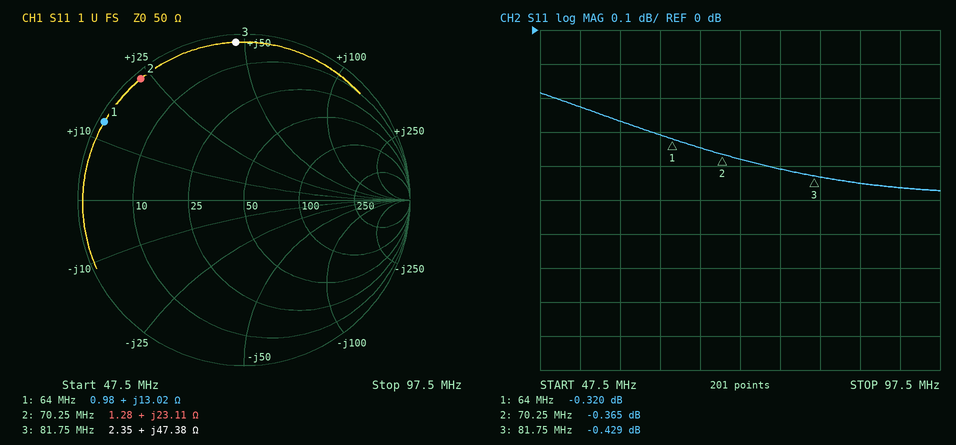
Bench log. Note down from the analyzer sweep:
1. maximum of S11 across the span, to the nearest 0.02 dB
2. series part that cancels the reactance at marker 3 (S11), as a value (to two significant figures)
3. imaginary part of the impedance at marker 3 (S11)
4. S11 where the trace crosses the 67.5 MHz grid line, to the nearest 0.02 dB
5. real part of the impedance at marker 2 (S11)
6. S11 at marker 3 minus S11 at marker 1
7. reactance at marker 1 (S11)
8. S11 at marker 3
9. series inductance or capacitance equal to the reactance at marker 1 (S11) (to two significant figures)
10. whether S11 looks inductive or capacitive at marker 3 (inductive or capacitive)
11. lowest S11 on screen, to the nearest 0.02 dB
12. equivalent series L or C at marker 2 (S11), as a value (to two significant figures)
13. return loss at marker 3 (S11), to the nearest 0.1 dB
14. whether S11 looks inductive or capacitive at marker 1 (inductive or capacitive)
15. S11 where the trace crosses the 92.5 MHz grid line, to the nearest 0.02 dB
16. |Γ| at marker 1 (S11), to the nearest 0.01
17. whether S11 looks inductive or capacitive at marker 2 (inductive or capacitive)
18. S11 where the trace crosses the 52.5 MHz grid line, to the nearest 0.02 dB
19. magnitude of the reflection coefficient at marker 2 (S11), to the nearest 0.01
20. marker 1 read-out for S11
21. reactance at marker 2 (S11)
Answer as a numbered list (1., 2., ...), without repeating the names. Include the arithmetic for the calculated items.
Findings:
1. -0.18 dB
2. C = 1/(2π × 81.75 MHz × 47.38 Ω) ≈ 41 pF
3. +47.38 Ω
4. -0.34 dB
5. 1.28 Ω
6. -0.429 − (-0.32) = -0.109 dB
7. +13.02 Ω
8. -0.429 dB
9. L = 13.02 Ω/(2π × 64 MHz) ≈ 32 nH
10. inductive
11. -0.48 dB
12. L = 23.11 Ω/(2π × 70.25 MHz) ≈ 52 nH
13. 0.4 dB
14. inductive
15. -0.46 dB
16. 0.96
17. inductive
18. -0.22 dB
19. 0.96
20. -0.320 dB
21. +23.11 Ω
